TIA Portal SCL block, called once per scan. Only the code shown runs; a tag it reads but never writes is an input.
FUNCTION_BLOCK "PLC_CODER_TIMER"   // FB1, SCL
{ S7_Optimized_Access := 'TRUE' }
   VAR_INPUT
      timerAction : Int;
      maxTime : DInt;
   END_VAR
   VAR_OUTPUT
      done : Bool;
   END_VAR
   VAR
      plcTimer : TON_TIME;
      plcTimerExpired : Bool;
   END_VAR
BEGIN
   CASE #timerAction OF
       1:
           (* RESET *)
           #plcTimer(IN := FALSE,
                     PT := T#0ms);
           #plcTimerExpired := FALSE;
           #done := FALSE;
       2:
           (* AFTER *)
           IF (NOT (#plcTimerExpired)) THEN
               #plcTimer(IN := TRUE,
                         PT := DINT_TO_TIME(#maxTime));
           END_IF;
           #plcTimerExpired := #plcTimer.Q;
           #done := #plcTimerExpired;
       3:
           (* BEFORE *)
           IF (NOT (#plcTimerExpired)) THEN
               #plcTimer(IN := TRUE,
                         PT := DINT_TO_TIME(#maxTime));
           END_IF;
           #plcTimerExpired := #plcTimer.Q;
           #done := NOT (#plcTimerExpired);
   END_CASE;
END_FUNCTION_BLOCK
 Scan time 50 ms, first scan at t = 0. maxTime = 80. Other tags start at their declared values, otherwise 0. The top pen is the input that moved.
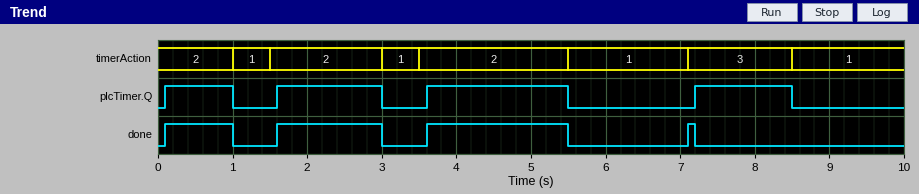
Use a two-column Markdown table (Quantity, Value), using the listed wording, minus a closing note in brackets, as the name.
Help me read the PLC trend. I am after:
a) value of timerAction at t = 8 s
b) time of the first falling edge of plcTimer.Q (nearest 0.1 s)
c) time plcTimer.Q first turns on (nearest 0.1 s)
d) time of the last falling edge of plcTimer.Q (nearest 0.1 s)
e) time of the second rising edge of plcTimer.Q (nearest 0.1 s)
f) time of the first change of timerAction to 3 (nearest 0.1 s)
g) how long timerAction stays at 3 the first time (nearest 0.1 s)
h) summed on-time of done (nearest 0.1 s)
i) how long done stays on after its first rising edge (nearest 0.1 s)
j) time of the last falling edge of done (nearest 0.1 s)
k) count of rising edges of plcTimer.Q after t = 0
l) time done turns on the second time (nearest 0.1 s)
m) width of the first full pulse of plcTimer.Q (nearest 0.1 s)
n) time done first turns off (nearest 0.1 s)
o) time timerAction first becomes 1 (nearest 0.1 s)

| Quantity | Value |
|---|---|
| value of timerAction at t = 8 s | 3 |
| time of the first falling edge of plcTimer.Q | 1.0 s |
| time plcTimer.Q first turns on | 0.1 s |
| time of the last falling edge of plcTimer.Q | 8.5 s |
| time of the second rising edge of plcTimer.Q | 1.6 s |
| time of the first change of timerAction to 3 | 7.1 s |
| how long timerAction stays at 3 the first time | 1.4 s |
| summed on-time of done | 4.3 s |
| how long done stays on after its first rising edge | 0.9 s |
| time of the last falling edge of done | 7.2 s |
| count of rising edges of plcTimer.Q after t = 0 | 4 |
| time done turns on the second time | 1.6 s |
| width of the first full pulse of plcTimer.Q | 0.9 s |
| time done first turns off | 1.0 s |
| time timerAction first becomes 1 | 1.0 s |
